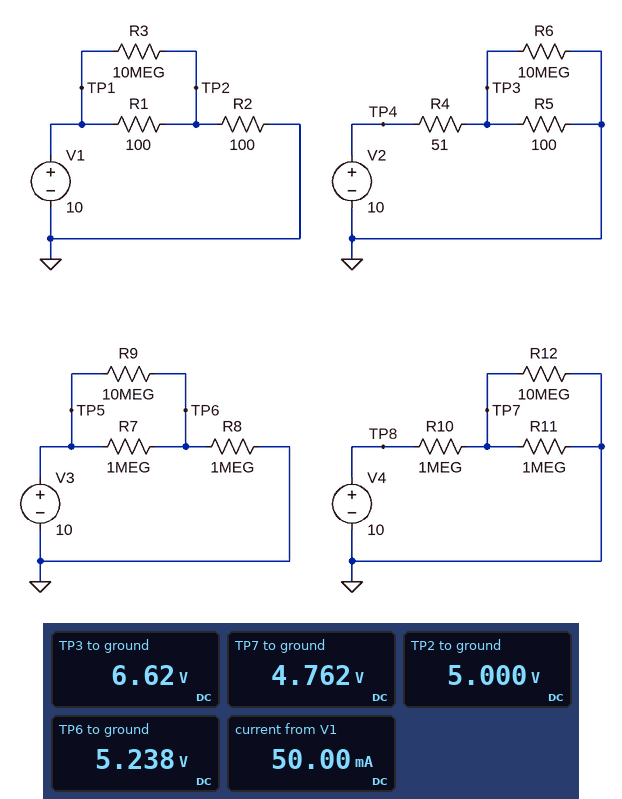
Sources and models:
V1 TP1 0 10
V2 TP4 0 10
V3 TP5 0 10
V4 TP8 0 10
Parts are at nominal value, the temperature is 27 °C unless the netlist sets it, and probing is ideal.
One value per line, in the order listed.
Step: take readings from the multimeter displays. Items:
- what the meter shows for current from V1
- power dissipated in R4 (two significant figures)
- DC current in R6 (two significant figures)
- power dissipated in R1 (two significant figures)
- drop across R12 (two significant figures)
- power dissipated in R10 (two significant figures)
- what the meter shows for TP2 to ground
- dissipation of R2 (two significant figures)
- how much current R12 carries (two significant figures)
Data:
50.00 mA
220 mW
660 nA
250 mW
4.8 V
27 µW
5.000 V
250 mW
480 nA
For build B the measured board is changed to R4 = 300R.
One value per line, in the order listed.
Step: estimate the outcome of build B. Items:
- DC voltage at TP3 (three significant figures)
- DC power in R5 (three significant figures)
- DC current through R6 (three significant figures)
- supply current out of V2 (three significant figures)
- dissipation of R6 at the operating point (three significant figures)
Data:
2.50 V
62.5 mW
250 nA
25.0 mA
625 nW
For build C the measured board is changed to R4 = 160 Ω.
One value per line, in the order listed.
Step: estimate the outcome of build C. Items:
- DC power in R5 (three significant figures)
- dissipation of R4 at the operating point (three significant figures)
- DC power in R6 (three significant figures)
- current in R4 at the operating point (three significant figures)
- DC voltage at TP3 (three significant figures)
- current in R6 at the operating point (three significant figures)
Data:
148 mW
237 mW
1.48 µW
38.5 mA
3.85 V
385 nA
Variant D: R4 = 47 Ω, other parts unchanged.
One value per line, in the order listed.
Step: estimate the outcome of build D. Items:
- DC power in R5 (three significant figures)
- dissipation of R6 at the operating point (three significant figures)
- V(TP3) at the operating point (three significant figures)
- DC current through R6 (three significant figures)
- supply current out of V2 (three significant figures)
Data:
463 mW
4.63 µW
6.80 V
680 nA
68.0 mA
